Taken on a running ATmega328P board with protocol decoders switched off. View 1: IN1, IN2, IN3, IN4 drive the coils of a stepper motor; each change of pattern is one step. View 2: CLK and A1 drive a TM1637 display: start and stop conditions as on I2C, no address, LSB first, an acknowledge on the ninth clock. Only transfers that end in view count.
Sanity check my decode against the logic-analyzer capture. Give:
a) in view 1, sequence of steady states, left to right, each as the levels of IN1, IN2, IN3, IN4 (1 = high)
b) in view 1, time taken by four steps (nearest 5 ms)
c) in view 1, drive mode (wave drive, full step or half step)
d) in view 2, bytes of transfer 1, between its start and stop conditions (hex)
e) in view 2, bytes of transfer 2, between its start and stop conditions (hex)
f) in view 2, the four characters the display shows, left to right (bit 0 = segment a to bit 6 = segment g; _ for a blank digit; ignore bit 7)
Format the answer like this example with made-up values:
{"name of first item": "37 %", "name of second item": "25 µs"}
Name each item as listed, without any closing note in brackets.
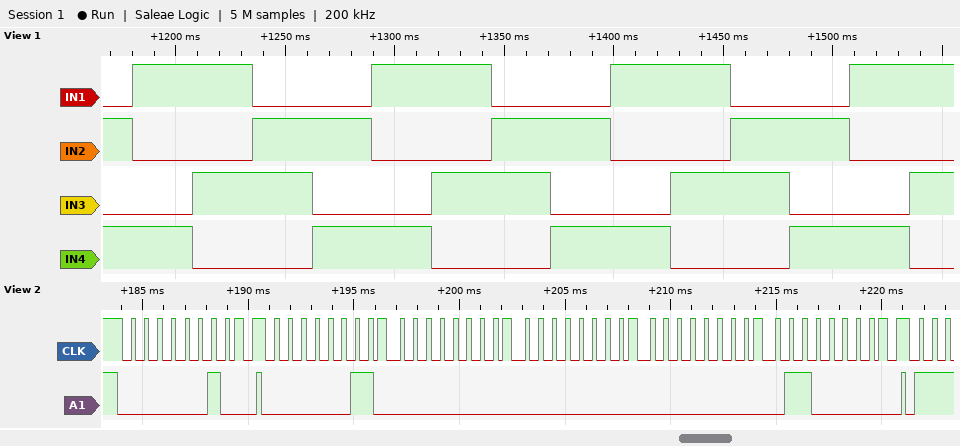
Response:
{"in view 1, sequence of steady states, left to right, each as the levels of IN1, IN2, IN3, IN4": "0101 1001 1010 0110 0101 1001 1010 0110 0101 1001 1010 0110 0101 1001 1010", "in view 1, time taken by four steps": "110 ms", "in view 1, drive mode": "full step", "in view 2, bytes of transfer 1, between its start and stop conditions": "40", "in view 2, bytes of transfer 2, between its start and stop conditions": "C0 00 00 00 06", "in view 2, the four characters the display shows, left to right": "___1"}
